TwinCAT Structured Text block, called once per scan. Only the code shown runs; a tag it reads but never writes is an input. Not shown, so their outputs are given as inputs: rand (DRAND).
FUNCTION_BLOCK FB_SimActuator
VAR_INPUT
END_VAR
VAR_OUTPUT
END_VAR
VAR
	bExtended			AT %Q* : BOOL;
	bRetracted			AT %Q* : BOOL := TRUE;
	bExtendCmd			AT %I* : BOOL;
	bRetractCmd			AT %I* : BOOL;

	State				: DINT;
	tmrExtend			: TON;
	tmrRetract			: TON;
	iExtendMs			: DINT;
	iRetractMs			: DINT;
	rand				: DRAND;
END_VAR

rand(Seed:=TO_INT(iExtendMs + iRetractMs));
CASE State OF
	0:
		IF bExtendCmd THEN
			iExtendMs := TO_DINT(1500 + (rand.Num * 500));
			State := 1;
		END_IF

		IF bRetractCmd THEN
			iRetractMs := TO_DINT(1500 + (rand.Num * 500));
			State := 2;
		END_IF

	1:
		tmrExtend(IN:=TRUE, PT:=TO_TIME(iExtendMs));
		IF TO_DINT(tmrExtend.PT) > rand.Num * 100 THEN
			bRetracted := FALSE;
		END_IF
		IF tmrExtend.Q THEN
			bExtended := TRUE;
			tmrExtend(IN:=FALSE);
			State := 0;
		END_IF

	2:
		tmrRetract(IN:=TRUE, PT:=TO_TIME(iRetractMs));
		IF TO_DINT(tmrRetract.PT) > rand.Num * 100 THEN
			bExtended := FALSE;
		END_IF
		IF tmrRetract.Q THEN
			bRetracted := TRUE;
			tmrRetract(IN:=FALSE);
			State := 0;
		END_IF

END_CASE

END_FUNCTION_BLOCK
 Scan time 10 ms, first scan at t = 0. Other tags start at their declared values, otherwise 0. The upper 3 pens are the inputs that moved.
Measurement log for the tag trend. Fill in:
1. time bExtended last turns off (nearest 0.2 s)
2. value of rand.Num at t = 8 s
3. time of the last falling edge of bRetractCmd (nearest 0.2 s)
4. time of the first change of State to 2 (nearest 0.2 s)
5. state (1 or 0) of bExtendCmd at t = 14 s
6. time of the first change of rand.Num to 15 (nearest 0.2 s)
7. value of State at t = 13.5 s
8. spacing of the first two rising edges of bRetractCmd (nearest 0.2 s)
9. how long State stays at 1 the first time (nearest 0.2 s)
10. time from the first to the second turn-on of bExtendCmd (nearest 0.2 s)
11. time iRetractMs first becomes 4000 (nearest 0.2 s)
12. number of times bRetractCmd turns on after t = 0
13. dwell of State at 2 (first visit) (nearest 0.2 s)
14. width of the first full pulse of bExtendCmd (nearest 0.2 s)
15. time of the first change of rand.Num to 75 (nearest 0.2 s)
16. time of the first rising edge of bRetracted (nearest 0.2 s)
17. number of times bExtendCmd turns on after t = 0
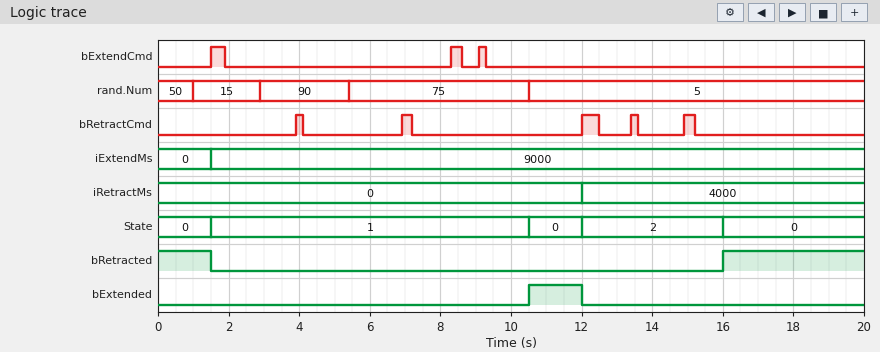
12.0 s
75
15.2 s
12.0 s
0
1.0 s
2
3.0 s
9.0 s
6.8 s
12.0 s
5
4.0 s
0.4 s
5.4 s
16.0 s
3
